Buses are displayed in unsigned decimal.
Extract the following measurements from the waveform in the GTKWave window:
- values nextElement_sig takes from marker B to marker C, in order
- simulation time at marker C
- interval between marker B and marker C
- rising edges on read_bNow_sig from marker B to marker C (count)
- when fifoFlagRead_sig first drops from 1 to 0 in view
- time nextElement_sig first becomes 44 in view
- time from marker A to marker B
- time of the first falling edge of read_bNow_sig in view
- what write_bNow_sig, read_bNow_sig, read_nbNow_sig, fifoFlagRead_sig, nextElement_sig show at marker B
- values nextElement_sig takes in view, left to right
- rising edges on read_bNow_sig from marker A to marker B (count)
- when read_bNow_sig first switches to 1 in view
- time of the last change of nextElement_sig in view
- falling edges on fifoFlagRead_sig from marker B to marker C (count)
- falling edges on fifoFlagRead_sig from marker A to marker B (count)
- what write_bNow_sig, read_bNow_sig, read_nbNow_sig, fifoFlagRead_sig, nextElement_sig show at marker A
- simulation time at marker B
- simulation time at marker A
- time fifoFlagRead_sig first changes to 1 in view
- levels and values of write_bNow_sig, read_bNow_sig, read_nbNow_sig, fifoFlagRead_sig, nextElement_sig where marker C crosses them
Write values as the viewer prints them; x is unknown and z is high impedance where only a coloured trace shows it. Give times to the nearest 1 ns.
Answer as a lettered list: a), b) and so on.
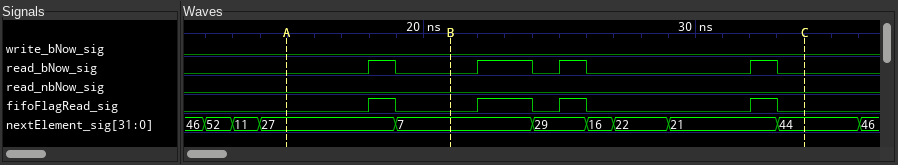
a) 7, 29, 16, 22, 21, 44
b) 34 ns
c) 13 ns
d) 3
e) 19 ns
f) 33 ns
g) 6 ns
h) 19 ns
i) write_bNow_sig=0, read_bNow_sig=0, read_nbNow_sig=0, fifoFlagRead_sig=0, nextElement_sig=7
j) 46, 52, 11, 27, 7, 29, 16, 22, 21, 44, 46
k) 1
l) 18 ns
m) 36 ns
n) 3
o) 1
p) write_bNow_sig=0, read_bNow_sig=0, read_nbNow_sig=0, fifoFlagRead_sig=0, nextElement_sig=27
q) 21 ns
r) 15 ns
s) 18 ns
t) write_bNow_sig=0, read_bNow_sig=0, read_nbNow_sig=0, fifoFlagRead_sig=0, nextElement_sig=44
